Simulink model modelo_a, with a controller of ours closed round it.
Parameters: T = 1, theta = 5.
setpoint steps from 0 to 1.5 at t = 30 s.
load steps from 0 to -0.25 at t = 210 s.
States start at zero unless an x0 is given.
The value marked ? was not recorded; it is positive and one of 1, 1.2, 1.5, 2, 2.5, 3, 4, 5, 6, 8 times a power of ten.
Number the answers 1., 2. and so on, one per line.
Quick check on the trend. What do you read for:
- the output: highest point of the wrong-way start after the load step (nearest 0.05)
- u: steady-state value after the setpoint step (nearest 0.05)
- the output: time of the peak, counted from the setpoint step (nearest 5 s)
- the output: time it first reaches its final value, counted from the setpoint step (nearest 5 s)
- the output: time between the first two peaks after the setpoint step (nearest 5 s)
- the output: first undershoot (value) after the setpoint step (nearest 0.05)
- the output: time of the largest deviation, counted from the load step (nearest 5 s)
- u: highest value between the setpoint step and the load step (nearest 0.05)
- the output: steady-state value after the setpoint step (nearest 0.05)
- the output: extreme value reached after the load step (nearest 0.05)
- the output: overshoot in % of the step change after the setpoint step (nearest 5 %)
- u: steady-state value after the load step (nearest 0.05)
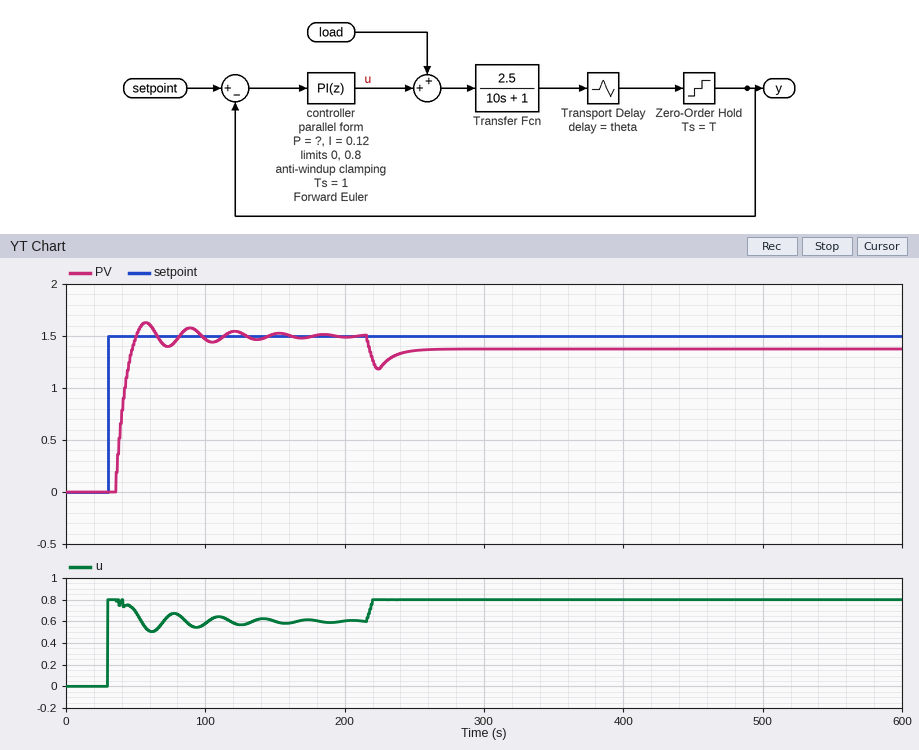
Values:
1. 1.50
2. 0.60
3. 25 s
4. 20 s
5. 30 s
6. 1.40
7. 15 s
8. 0.80
9. 1.50
10. 1.20
11. 10 %
12. 0.80
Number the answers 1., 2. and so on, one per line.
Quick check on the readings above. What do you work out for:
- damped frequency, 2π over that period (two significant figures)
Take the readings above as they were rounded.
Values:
1. 0.21 rad/s
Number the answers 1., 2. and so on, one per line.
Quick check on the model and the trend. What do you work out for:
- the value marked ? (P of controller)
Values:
1. 0.6
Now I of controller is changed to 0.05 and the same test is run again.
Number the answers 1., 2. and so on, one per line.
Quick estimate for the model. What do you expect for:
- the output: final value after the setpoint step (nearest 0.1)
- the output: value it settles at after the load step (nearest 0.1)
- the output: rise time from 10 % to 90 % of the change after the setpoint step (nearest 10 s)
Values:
1. 1.5
2. 1.4
3. 30 s
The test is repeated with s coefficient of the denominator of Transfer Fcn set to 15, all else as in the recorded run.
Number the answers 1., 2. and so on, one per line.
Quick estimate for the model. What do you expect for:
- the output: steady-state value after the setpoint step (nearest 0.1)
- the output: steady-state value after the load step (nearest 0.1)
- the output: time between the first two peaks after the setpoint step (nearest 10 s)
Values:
1. 1.5
2. 1.4
3. 40 s
